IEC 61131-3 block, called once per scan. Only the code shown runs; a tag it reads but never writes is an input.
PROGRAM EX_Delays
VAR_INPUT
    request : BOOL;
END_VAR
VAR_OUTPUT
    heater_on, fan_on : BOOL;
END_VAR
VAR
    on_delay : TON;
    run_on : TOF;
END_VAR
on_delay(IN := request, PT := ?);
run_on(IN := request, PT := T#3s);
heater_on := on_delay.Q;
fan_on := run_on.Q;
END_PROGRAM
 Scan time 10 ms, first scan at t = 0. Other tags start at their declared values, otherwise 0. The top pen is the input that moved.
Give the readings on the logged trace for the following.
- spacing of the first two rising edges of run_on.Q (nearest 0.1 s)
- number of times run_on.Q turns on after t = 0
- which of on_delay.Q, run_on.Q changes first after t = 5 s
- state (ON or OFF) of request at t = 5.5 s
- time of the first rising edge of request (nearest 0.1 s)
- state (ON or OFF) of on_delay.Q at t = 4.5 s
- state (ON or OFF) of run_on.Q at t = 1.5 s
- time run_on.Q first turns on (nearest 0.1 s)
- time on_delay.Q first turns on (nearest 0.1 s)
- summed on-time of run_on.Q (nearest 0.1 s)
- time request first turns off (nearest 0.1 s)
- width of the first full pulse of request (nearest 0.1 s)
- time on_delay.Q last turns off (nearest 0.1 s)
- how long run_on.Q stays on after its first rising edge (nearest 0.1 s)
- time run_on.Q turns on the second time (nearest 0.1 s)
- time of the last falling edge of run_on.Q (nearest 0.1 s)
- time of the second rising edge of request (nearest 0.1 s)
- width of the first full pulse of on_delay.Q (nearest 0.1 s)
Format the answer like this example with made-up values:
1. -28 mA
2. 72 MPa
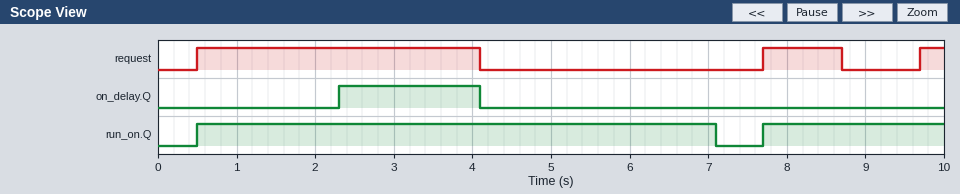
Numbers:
1. 7.2 s
2. 2
3. run_on.Q
4. OFF
5. 0.5 s
6. OFF
7. ON
8. 0.5 s
9. 2.3 s
10. 8.9 s
11. 4.1 s
12. 3.6 s
13. 4.1 s
14. 6.6 s
15. 7.7 s
16. 7.1 s
17. 7.7 s
18. 1.8 s
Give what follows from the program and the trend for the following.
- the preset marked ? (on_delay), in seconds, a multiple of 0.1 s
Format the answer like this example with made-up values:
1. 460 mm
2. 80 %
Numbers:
1. 1.8 s
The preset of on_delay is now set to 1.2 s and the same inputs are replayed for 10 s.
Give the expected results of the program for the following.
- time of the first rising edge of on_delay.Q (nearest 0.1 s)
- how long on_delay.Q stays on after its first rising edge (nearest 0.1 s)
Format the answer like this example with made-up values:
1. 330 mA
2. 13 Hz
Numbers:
1. 1.7 s
2. 2.4 s
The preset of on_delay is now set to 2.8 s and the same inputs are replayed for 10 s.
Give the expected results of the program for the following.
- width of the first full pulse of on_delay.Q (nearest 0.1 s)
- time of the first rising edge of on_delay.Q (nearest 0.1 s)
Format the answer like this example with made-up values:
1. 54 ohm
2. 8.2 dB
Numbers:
1. 0.8 s
2. 3.3 s
